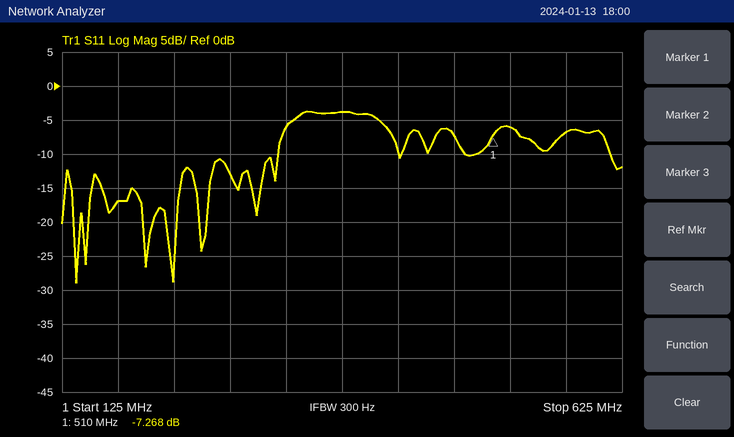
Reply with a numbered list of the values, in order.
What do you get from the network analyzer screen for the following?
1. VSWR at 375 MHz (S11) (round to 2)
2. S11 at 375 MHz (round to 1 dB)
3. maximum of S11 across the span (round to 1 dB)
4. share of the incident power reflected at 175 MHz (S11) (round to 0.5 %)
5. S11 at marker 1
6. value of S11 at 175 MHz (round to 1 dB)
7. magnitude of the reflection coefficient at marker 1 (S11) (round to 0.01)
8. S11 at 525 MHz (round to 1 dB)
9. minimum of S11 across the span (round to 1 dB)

1. 4
2. -4 dB
3. -4 dB
4. 2.0 %
5. -7.268 dB
6. -17 dB
7. 0.43
8. -6 dB
9. -29 dB
